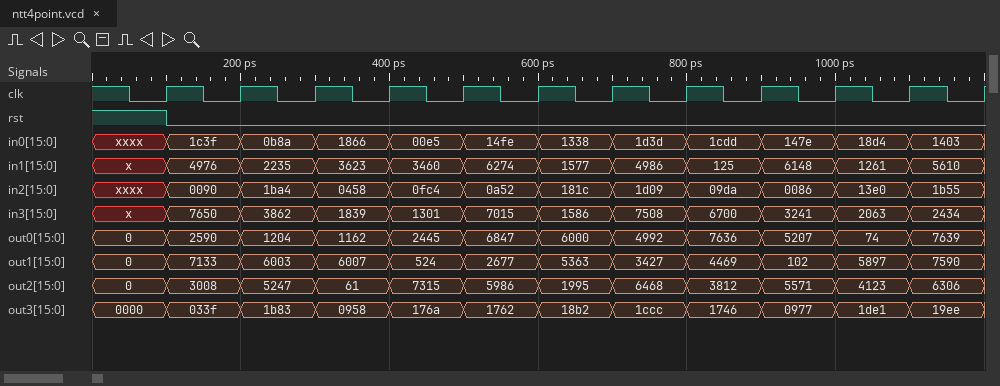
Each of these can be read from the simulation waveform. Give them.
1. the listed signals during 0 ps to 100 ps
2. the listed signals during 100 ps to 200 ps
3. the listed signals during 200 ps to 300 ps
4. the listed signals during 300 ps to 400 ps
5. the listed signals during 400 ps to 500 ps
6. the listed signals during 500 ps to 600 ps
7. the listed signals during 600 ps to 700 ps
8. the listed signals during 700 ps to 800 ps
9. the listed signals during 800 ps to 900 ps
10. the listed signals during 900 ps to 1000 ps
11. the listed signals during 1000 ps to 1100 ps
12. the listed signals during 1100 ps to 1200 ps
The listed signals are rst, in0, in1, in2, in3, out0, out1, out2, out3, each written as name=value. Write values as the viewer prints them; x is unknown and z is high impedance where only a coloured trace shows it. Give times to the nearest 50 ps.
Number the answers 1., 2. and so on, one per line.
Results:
1. rst=1, in0=xxxx, in1=x, in2=xxxx, in3=x, out0=0, out1=0, out2=0, out3=0000
2. rst=0, in0=1c3f, in1=4976, in2=0090, in3=7650, out0=2590, out1=7133, out2=3008, out3=033f
3. rst=0, in0=0b8a, in1=2235, in2=1ba4, in3=3862, out0=1204, out1=6003, out2=5247, out3=1b83
4. rst=0, in0=1866, in1=3623, in2=0458, in3=1839, out0=1162, out1=6007, out2=61, out3=0958
5. rst=0, in0=00e5, in1=3460, in2=0fc4, in3=1301, out0=2445, out1=524, out2=7315, out3=176a
6. rst=0, in0=14fe, in1=6274, in2=0a52, in3=7015, out0=6847, out1=2677, out2=5986, out3=1762
7. rst=0, in0=1338, in1=1577, in2=181c, in3=1586, out0=6000, out1=5363, out2=1995, out3=18b2
8. rst=0, in0=1d3d, in1=4986, in2=1d09, in3=7508, out0=4992, out1=3427, out2=6468, out3=1ccc
9. rst=0, in0=1cdd, in1=125, in2=09da, in3=6700, out0=7636, out1=4469, out2=3812, out3=1746
10. rst=0, in0=147e, in1=6148, in2=0086, in3=3241, out0=5207, out1=102, out2=5571, out3=0977
11. rst=0, in0=18d4, in1=1261, in2=13e0, in3=2063, out0=74, out1=5897, out2=4123, out3=1de1
12. rst=0, in0=1403, in1=5610, in2=1b55, in3=2434, out0=7639, out1=7590, out2=6306, out3=19ee
